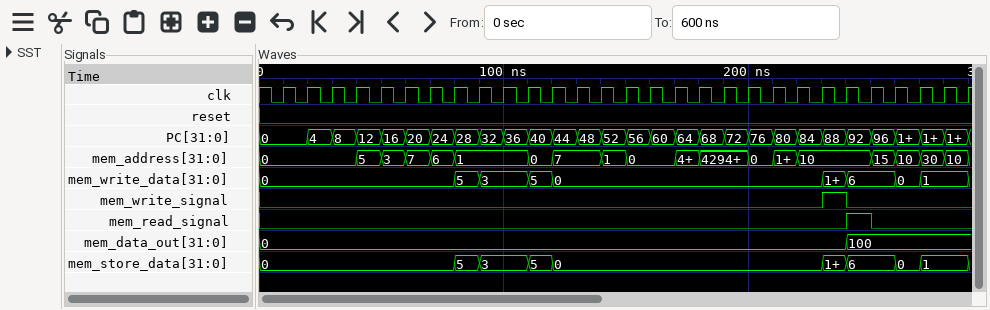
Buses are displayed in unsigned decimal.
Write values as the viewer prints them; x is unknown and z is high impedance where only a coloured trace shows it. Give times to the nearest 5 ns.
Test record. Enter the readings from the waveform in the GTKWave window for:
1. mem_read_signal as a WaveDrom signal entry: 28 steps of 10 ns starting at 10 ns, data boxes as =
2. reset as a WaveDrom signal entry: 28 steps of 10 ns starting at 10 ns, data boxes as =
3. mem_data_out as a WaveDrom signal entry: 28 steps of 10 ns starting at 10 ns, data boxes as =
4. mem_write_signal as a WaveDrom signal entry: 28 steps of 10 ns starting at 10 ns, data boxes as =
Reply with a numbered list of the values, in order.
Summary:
1. {name: 'mem_read_signal', wave: '0......................10...'}
2. {name: 'reset', wave: '0...........................'}
3. {name: 'mem_data_out', wave: '=......................=....', data: '0 100'}
4. {name: 'mem_write_signal', wave: '0.....................10....'}
